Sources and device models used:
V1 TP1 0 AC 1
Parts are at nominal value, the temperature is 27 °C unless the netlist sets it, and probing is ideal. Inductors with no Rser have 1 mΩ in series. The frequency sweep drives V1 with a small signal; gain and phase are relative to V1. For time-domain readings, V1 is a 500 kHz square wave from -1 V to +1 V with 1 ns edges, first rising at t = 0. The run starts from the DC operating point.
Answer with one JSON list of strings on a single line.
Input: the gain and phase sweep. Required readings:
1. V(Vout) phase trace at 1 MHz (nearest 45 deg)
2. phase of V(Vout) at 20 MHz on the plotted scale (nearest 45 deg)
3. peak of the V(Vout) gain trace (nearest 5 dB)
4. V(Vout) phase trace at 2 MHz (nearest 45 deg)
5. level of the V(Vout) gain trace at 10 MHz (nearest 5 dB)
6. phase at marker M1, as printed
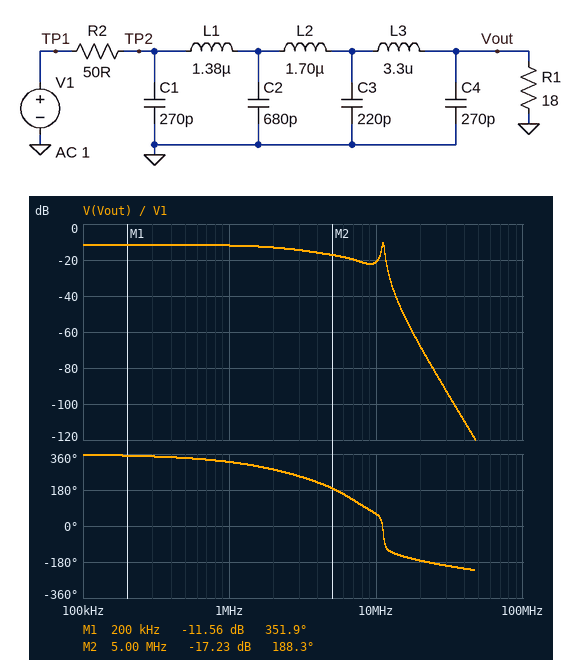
["315 deg", "-180 deg", "-10 dB", "270 deg", "-20 dB", "351.9 deg"]
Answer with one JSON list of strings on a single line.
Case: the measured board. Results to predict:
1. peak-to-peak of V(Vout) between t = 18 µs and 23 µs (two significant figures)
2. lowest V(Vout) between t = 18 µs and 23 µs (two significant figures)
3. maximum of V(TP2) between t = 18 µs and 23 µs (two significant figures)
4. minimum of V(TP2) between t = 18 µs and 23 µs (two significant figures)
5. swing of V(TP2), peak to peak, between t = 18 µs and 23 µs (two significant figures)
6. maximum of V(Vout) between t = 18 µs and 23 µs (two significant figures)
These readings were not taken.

["550 mV", "-280 mV", "1.2 V", "-1.2 V", "2.3 V", "280 mV"]
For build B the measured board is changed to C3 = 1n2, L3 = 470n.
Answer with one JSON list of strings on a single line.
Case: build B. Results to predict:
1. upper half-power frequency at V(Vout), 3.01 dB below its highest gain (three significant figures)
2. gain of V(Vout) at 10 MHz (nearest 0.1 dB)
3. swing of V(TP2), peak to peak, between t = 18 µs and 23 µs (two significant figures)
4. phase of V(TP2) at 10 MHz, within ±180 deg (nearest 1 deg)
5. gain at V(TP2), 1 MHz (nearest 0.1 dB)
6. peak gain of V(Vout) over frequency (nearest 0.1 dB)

["8.51 MHz", "-22.7 dB", "2.1 V", "3 deg", "-8.4 dB", "-11.1 dB"]
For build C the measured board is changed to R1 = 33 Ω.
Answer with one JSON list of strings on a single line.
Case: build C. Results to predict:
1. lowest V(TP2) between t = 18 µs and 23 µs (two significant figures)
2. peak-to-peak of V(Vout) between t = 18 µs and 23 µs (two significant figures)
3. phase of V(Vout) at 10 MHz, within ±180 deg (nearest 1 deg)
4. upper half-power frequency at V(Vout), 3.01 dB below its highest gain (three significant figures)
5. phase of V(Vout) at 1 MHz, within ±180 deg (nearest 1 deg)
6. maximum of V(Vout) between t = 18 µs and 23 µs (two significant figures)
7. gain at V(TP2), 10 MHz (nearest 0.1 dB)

["-1.0 V", "840 mV", "48 deg", "11.4 MHz", "-38 deg", "420 mV", "-0.5 dB"]
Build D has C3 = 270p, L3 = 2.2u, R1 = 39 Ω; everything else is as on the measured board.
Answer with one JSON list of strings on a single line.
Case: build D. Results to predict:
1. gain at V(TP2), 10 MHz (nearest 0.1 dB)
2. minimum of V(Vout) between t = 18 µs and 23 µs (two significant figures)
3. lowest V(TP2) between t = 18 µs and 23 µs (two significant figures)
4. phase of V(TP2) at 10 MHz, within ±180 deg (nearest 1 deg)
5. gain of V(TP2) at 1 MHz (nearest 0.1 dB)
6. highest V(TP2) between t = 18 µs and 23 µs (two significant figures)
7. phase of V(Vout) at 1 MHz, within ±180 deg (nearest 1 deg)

["-1.0 dB", "-470 mV", "-880 mV", "-11 deg", "-5.7 dB", "880 mV", "-33 deg"]
